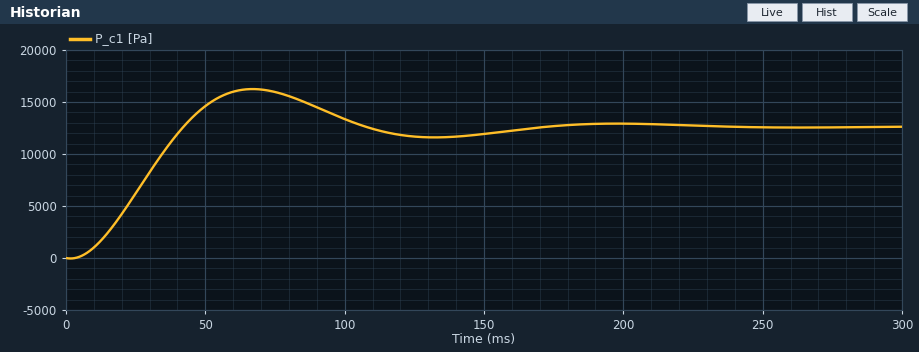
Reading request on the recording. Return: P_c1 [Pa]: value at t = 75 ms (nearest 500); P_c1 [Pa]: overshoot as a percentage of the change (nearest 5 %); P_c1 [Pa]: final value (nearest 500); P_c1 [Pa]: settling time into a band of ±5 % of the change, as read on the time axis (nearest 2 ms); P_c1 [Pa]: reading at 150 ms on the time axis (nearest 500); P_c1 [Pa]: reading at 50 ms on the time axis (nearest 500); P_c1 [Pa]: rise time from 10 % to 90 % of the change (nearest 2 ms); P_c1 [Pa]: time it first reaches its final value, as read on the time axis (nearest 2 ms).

16000
30 %
12500
152 ms
12000
14500
28 ms
42 ms
